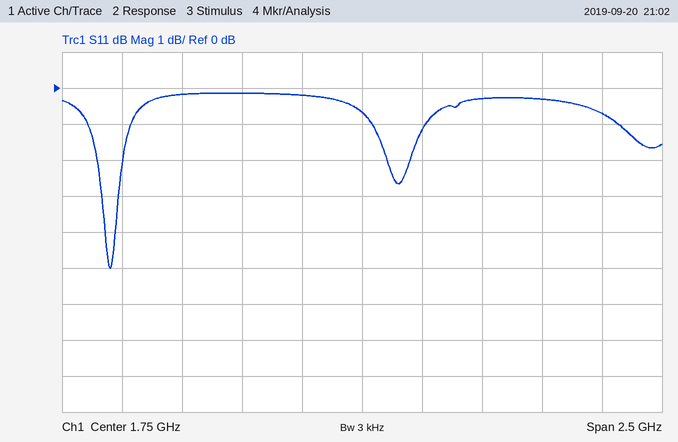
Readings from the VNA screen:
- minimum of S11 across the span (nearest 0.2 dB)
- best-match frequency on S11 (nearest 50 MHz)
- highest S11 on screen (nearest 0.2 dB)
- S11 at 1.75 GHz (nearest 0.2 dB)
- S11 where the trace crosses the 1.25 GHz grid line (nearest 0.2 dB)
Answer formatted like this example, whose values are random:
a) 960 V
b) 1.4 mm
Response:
a) -5.0 dB
b) 700 MHz
c) -0.2 dB
d) -0.6 dB
e) -0.2 dB
